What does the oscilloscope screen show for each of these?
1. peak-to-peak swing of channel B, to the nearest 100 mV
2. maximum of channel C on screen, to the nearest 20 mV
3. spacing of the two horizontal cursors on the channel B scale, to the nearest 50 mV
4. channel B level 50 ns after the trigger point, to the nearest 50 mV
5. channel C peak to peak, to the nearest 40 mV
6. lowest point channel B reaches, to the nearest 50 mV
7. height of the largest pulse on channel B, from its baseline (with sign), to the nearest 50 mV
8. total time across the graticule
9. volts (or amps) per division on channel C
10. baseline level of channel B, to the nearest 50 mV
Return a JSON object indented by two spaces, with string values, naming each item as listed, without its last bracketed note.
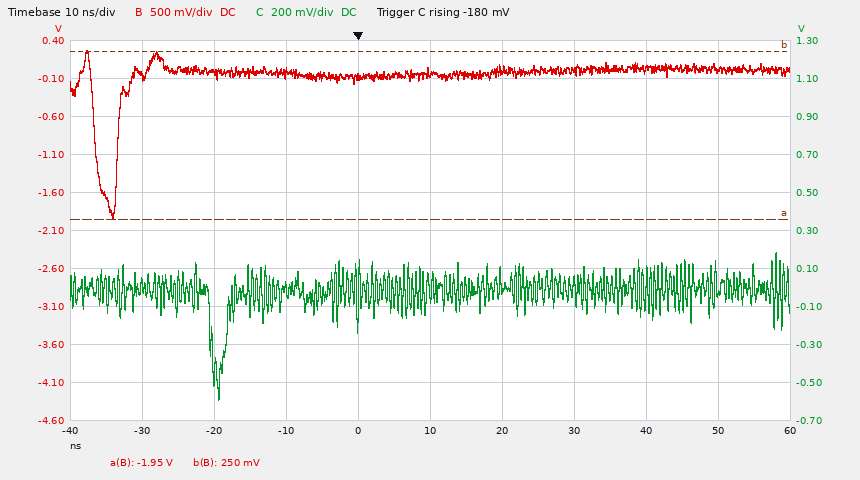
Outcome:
{
  "peak-to-peak swing of channel B, to the nearest 100 mV": "2.20 V",
  "maximum of channel C on screen, to the nearest 20 mV": "180 mV",
  "spacing of the two horizontal cursors on the channel B scale, to the nearest 50 mV": "2.20 V",
  "channel B level 50 ns after the trigger point, to the nearest 50 mV": "0 mV",
  "channel C peak to peak, to the nearest 40 mV": "760 mV",
  "lowest point channel B reaches, to the nearest 50 mV": "-1.95 V",
  "height of the largest pulse on channel B, from its baseline (with sign), to the nearest 50 mV": "-1.95 V",
  "total time across the graticule": "100 ns",
  "volts (or amps) per division on channel C": "200 mV",
  "baseline level of channel B, to the nearest 50 mV": "0 mV"
}
